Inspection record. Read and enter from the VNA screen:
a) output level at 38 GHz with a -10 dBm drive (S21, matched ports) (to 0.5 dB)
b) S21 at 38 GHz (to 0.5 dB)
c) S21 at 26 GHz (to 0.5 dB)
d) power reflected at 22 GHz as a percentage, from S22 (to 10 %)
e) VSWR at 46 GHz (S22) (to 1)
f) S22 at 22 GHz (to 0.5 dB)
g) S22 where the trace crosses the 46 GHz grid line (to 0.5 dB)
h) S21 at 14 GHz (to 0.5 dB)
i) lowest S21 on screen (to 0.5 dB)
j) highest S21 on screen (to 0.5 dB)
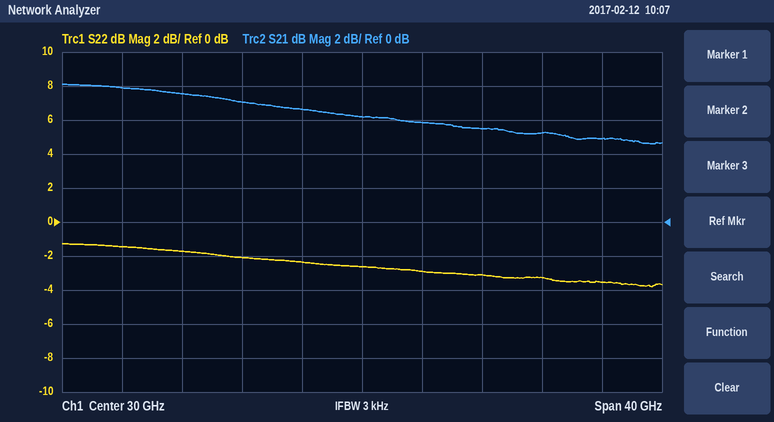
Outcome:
-4.5 dBm
5.5 dB
6.5 dB
60 %
5
-2.0 dB
-3.5 dB
8.0 dB
4.5 dB
8.0 dB
